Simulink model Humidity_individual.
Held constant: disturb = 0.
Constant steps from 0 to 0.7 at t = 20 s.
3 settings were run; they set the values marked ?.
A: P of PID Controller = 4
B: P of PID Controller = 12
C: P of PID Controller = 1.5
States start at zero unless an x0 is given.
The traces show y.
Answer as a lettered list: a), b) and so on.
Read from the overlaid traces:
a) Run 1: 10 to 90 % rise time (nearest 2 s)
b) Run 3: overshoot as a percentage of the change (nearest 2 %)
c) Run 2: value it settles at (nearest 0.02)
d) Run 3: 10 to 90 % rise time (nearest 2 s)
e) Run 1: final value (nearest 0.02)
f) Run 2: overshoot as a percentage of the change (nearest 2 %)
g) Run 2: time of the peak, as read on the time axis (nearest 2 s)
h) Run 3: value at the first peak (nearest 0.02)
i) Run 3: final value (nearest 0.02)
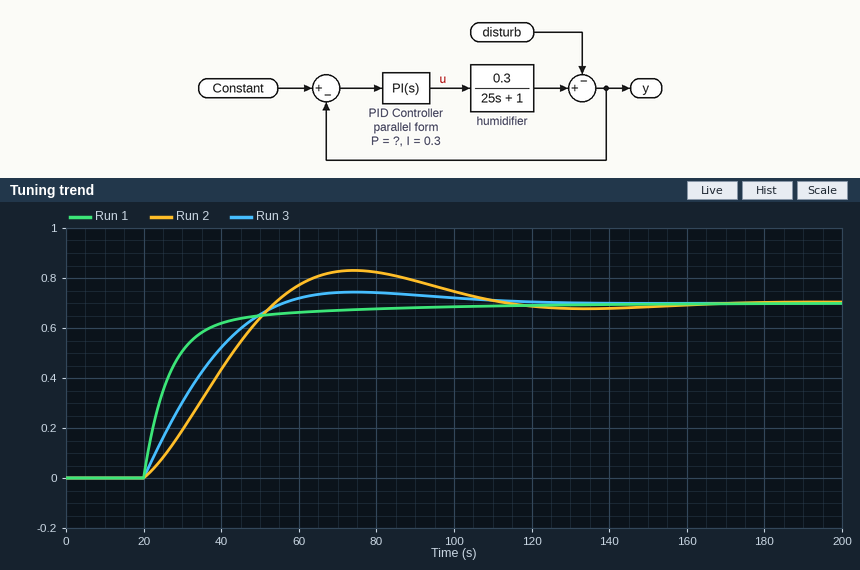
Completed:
a) 22 s
b) 6 %
c) 0.70
d) 26 s
e) 0.70
f) 18 %
g) 74 s
h) 0.74
i) 0.70
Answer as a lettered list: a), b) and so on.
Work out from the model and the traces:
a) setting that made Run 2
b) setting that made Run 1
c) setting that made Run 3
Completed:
a) C
b) B
c) A
